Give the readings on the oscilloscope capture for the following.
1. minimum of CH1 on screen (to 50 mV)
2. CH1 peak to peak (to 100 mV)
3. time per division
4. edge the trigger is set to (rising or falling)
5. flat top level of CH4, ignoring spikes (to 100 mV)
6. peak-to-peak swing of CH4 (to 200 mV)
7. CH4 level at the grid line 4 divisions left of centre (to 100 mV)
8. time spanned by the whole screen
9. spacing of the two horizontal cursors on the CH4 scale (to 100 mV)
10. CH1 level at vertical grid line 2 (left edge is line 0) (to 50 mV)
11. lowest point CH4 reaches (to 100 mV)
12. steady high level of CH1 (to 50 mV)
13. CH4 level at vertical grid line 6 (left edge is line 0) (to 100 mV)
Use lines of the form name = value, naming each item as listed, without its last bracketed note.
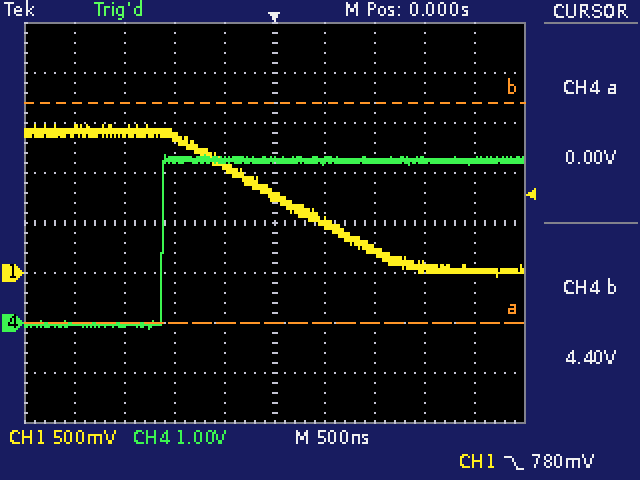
minimum of CH1 on screen = -50 mV
CH1 peak to peak = 1.50 V
time per division = 500 ns
edge the trigger is set to = falling
flat top level of CH4, ignoring spikes = 3.2 V
peak-to-peak swing of CH4 = 3.4 V
CH4 level at the grid line 4 divisions left of centre = 0.0 V
time spanned by the whole screen = 5 µs
spacing of the two horizontal cursors on the CH4 scale = 4.4 V
CH1 level at vertical grid line 2 (left edge is line 0) = 1.40 V
lowest point CH4 reaches = -100 mV
steady high level of CH1 = 1.40 V
CH4 level at vertical grid line 6 (left edge is line 0) = 3.2 V
